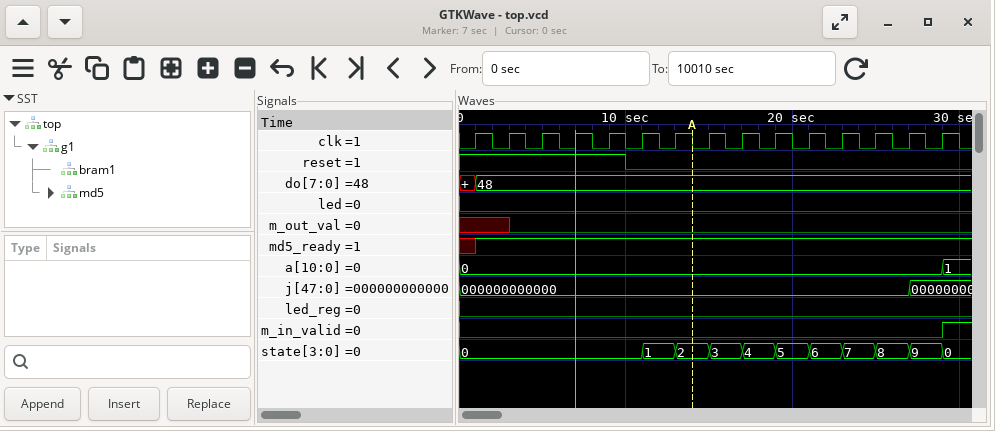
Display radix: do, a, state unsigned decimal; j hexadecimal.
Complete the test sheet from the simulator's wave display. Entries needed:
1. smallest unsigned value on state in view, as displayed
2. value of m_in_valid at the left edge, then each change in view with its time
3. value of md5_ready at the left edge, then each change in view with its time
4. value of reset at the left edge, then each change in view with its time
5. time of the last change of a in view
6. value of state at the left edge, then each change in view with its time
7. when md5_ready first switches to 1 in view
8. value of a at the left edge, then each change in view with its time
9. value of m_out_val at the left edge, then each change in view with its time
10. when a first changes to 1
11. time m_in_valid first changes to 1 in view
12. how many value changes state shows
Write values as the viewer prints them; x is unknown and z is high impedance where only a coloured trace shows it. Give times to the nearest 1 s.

0
0, 1 at 29 s
x, 1 at 1 s
1, 0 at 10 s
29 s
0, 1 at 11 s, 2 at 13 s, 3 at 15 s, 4 at 17 s, 5 at 19 s, 6 at 21 s, 7 at 23 s, 8 at 25 s, 9 at 27 s, 0 at 29 s
1 s
0, 1 at 29 s
x, 0 at 3 s
29 s
29 s
10
